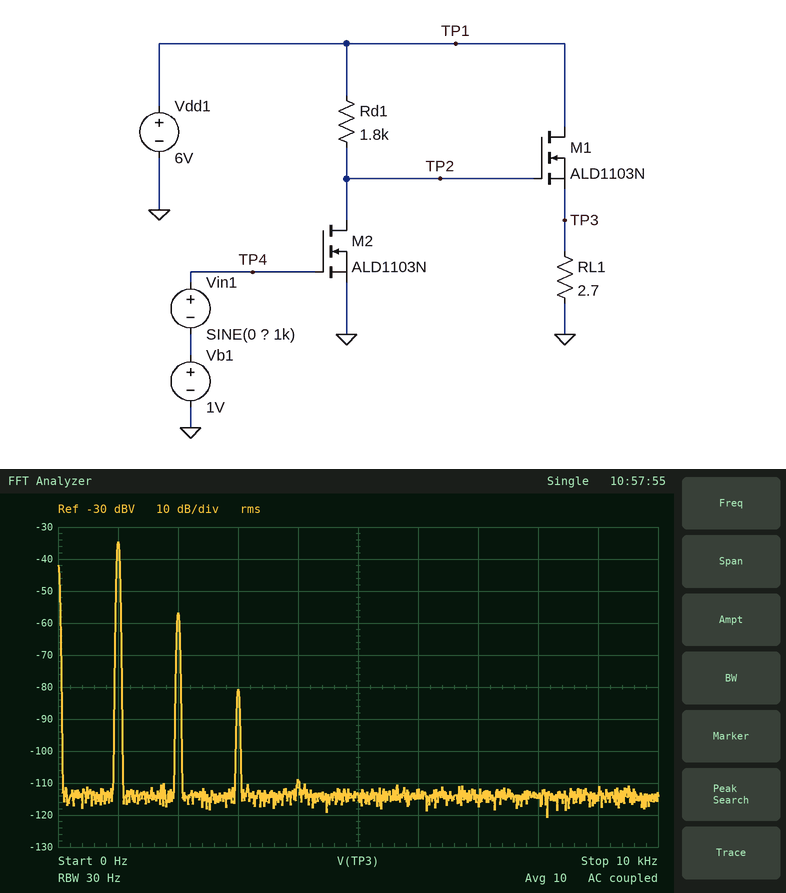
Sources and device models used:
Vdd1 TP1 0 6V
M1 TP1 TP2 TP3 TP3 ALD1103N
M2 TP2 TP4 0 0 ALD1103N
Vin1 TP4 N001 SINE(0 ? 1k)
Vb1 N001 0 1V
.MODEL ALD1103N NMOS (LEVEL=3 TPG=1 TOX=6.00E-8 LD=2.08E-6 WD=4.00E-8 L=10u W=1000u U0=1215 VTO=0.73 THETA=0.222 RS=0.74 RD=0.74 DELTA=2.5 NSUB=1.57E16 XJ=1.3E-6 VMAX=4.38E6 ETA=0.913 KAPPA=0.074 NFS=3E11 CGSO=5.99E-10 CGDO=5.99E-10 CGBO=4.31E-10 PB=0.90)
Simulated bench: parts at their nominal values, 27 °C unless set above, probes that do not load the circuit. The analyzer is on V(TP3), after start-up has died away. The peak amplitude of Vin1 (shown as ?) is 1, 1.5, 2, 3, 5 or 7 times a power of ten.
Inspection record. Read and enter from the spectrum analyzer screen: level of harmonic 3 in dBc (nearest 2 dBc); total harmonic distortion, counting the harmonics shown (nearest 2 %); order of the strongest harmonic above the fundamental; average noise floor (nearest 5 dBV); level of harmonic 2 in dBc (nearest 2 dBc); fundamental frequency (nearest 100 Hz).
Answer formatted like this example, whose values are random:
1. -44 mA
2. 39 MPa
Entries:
1. -46 dBc
2. 8 %
3. 2
4. -115 dBV
5. -22 dBc
6. 1.0 kHz
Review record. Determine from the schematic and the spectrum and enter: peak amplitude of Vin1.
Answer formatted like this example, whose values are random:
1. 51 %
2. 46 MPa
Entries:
1. 150 mV
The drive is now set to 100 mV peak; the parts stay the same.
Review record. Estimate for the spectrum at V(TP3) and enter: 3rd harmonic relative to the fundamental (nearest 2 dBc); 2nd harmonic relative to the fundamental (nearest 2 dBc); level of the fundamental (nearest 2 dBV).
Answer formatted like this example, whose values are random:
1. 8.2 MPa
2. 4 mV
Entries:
1. -54 dBc
2. -26 dBc
3. -38 dBV
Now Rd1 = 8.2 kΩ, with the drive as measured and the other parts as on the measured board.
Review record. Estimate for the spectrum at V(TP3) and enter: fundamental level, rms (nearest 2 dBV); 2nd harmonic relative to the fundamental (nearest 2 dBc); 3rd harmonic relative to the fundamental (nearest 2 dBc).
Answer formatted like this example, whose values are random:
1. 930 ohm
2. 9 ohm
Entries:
1. -28 dBV
2. -12 dBc
3. -22 dBc
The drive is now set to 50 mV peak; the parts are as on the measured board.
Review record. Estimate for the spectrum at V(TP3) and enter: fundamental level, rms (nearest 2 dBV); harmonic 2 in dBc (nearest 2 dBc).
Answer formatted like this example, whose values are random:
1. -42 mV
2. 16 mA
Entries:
1. -44 dBV
2. -32 dBc
